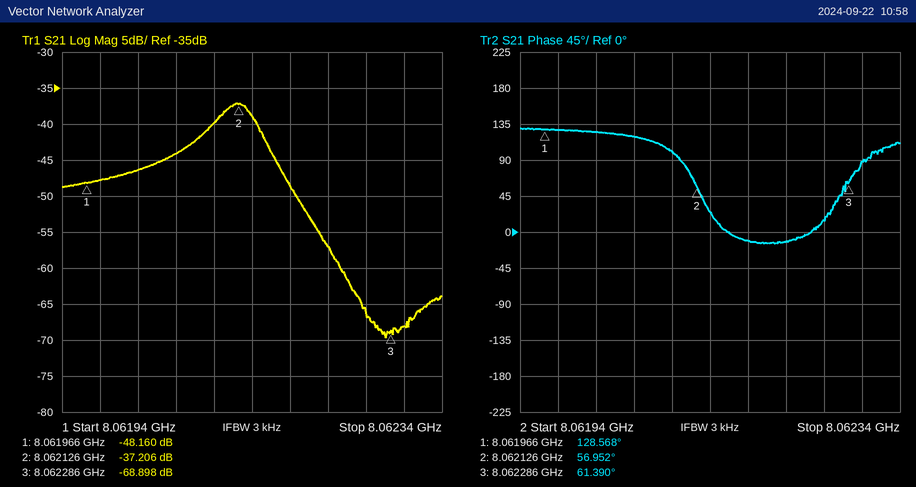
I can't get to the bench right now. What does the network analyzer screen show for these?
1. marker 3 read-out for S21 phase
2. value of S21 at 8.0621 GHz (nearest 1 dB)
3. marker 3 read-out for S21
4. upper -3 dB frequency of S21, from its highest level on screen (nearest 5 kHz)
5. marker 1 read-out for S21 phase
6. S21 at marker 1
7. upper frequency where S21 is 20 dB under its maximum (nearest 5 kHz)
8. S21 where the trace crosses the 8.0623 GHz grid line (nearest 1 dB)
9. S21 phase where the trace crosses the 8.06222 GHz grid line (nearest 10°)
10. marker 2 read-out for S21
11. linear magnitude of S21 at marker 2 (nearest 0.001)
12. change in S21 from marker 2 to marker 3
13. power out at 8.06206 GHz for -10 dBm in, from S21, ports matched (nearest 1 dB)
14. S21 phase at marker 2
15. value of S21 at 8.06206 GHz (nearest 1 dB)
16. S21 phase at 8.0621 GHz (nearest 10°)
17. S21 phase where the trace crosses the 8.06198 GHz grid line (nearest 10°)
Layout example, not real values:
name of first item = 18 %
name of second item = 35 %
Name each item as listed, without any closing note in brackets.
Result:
marker 3 read-out for S21 phase = 61.390°
value of S21 at 8.0621 GHz = -40 dB
marker 3 read-out for S21 = -68.898 dB
upper -3 dB frequency of S21, from its highest level on screen = 8.062145 GHz
marker 1 read-out for S21 phase = 128.568°
S21 at marker 1 = -48.160 dB
upper frequency where S21 is 20 dB under its maximum = 8.062220 GHz
S21 where the trace crosses the 8.0623 GHz grid line = -68 dB
S21 phase where the trace crosses the 8.06222 GHz grid line = -10°
marker 2 read-out for S21 = -37.206 dB
linear magnitude of S21 at marker 2 = 0.014
change in S21 from marker 2 to marker 3 = -31.692 dB
power out at 8.06206 GHz for -10 dBm in, from S21, ports matched = -54 dBm
S21 phase at marker 2 = 56.952°
value of S21 at 8.06206 GHz = -44 dB
S21 phase at 8.0621 GHz = 100°
S21 phase where the trace crosses the 8.06198 GHz grid line = 130°
